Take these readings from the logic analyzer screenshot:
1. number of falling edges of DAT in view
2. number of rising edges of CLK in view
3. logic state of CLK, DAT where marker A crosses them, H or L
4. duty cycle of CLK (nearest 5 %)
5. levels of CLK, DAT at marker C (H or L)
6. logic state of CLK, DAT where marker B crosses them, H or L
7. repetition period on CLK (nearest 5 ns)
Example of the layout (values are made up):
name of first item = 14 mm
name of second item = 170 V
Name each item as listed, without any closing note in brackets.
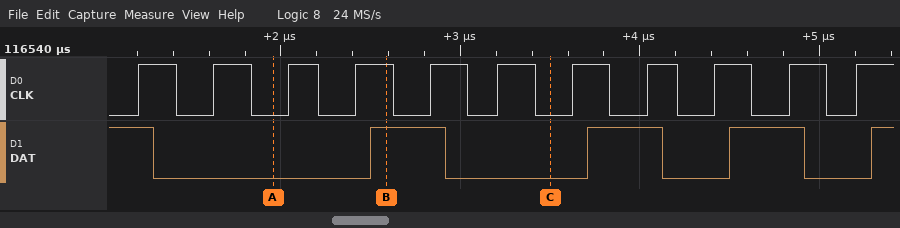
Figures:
number of falling edges of DAT in view = 4
number of rising edges of CLK in view = 11
logic state of CLK, DAT where marker A crosses them, H or L = CLK=L, DAT=L
duty cycle of CLK = 50 %
levels of CLK, DAT at marker C = CLK=L, DAT=L
logic state of CLK, DAT where marker B crosses them, H or L = CLK=H, DAT=H
repetition period on CLK = 400 ns
